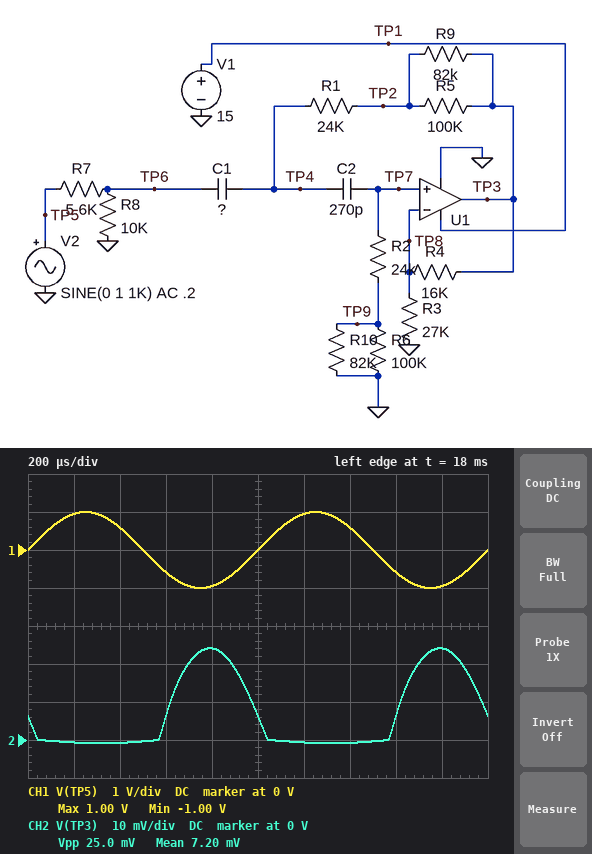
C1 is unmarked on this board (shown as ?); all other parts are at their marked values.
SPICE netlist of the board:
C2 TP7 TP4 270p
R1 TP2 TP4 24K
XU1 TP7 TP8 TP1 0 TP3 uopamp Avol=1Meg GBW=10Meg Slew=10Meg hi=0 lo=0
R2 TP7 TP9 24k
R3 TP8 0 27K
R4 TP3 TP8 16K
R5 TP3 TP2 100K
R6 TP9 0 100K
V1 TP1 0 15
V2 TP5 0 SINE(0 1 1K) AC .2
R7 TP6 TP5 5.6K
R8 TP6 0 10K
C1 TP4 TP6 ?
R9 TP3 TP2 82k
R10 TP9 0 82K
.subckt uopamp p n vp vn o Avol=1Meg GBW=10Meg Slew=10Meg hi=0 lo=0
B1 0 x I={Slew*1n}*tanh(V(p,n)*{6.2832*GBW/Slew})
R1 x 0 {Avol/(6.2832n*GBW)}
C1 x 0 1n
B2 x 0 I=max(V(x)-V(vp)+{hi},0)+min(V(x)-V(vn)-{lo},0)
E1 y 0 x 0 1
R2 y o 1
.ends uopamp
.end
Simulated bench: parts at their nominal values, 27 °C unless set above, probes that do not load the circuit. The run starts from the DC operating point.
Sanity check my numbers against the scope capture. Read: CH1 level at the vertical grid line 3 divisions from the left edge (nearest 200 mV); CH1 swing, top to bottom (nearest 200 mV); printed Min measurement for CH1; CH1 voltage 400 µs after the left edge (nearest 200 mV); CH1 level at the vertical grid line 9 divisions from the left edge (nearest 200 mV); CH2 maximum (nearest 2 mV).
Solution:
-600 mV
2.0 V
-1.00 V
600 mV
-1.0 V
24 mV
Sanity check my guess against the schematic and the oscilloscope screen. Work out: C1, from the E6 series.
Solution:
470 pF
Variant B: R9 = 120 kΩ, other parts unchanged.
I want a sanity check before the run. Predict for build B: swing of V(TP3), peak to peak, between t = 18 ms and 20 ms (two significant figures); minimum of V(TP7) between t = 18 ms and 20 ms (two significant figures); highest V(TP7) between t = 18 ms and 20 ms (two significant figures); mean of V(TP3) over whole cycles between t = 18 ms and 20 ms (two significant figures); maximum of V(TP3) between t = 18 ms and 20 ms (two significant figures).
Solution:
28 mV
-16 mV
17 mV
8.1 mV
27 mV
